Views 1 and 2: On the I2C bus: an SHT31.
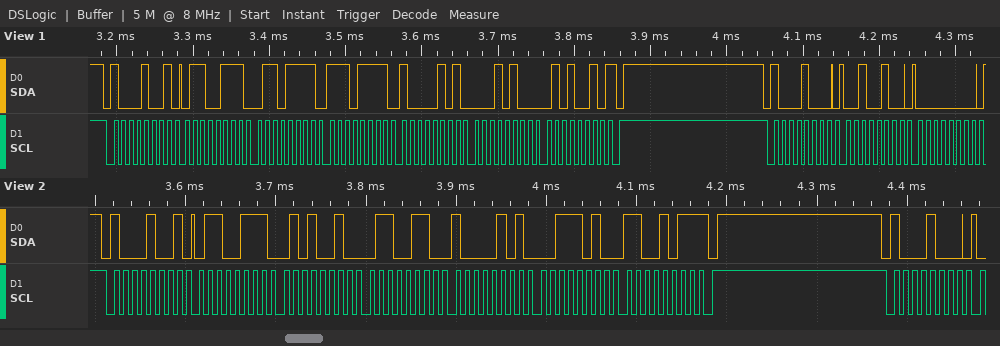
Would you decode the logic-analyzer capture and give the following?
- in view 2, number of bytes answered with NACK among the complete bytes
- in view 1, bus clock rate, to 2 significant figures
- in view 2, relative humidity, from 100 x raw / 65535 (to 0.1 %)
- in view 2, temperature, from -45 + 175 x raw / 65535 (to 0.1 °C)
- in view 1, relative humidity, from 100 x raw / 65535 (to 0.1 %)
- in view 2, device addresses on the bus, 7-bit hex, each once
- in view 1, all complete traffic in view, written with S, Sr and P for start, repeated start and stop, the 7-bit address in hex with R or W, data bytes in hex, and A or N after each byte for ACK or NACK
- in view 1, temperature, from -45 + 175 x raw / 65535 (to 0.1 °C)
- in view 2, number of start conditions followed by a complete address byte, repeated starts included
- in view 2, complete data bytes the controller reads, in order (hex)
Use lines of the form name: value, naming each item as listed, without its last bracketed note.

in view 2, number of bytes answered with NACK among the complete bytes: 1
in view 1, bus clock rate, to 2 significant figures: 100 kHz
in view 2, relative humidity, from 100 x raw / 65535: 52.0 %
in view 2, temperature, from -45 + 175 x raw / 65535: 25.6 °C
in view 1, relative humidity, from 100 x raw / 65535: 52.0 %
in view 2, device addresses on the bus, 7-bit hex, each once: 0x44
in view 1, all complete traffic in view, written with S, Sr and P for start, repeated start and stop, the 7-bit address in hex with R or W, data bytes in hex, and A or N after each byte for ACK or NACK: S 44R A 67 A 6F A EF A 85 A 14 A 52 N P S 44W A 24 A 00 A
in view 1, temperature, from -45 + 175 x raw / 65535: 25.7 °C
in view 2, number of start conditions followed by a complete address byte, repeated starts included: 2
in view 2, complete data bytes the controller reads, in order: 67 52 66 85 3A CB
